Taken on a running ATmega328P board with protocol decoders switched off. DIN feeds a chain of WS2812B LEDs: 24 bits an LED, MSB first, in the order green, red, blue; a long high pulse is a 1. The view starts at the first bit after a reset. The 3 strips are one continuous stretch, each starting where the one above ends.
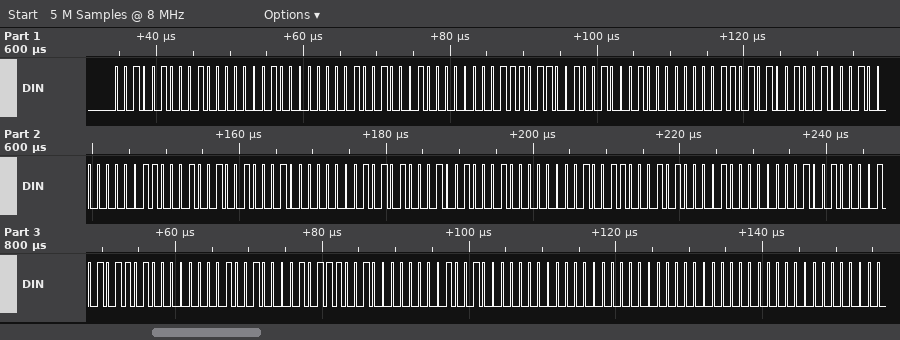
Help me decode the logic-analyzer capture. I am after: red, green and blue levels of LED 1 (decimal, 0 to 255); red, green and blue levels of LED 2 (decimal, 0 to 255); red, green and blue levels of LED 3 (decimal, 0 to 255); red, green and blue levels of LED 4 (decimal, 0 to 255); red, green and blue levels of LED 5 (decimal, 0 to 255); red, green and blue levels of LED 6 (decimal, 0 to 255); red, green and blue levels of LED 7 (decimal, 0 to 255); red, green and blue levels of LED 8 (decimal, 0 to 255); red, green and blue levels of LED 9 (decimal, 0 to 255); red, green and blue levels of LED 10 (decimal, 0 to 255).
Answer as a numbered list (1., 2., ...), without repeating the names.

1. 64, 36, 64
2. 64, 36, 59
3. 64, 36, 53
4. 64, 36, 49
5. 64, 36, 42
6. 64, 36, 38
7. 64, 40, 36
8. 64, 43, 36
9. 64, 46, 36
10. 0, 0, 0
